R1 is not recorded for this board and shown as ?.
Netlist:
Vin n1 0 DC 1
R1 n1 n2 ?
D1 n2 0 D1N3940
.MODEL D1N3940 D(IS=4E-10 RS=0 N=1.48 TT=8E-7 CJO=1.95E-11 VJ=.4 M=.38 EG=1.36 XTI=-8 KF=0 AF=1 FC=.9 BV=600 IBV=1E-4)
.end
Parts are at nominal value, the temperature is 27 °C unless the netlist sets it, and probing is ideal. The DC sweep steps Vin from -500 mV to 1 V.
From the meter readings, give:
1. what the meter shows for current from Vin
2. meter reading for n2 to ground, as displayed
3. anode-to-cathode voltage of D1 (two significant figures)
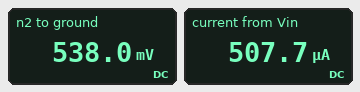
507.7 µA
538.0 mV
540 mV
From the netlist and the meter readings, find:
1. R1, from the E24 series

910 Ω
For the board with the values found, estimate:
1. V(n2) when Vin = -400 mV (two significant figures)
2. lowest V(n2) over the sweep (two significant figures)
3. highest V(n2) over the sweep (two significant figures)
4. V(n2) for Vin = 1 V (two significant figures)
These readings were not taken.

-400 mV
-500 mV
540 mV
540 mV
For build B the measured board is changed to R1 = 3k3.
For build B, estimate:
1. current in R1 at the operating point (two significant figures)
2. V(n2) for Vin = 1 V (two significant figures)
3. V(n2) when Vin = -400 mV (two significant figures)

150 µA
490 mV
-400 mV
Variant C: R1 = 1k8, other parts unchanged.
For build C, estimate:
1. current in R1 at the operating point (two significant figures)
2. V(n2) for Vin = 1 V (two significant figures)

270 µA
510 mV
